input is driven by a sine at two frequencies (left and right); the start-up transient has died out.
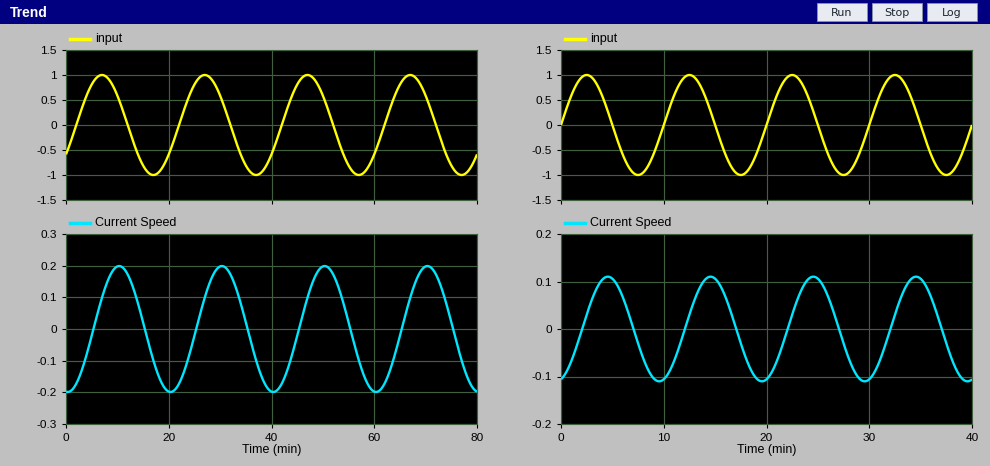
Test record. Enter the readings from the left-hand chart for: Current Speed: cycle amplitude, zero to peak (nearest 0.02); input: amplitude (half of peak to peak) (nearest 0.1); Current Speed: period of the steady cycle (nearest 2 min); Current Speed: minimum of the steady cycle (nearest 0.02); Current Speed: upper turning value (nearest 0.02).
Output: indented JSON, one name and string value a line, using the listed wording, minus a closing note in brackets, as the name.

{
  "Current Speed: cycle amplitude, zero to peak": "0.20",
  "input: amplitude (half of peak to peak)": "1.0",
  "Current Speed: period of the steady cycle": "20 min",
  "Current Speed: minimum of the steady cycle": "-0.20",
  "Current Speed: upper turning value": "0.20"
}
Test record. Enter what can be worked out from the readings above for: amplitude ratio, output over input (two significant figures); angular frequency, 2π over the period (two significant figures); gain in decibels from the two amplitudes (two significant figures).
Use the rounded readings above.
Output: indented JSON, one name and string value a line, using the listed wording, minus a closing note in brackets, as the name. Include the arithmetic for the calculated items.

{
  "amplitude ratio, output over input": "0.2 / 1 = 0.20",
  "angular frequency, 2π over the period": "2π / 20 = 0.31 rad/min",
  "gain in decibels from the two amplitudes": "20 log10(0.2 / 1) = -14 dB"
}
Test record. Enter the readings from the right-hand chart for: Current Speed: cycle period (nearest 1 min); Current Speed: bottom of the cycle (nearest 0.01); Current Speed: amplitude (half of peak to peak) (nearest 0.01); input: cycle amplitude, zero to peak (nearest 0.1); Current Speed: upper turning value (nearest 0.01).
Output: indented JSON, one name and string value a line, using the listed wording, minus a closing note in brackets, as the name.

{
  "Current Speed: cycle period": "10 min",
  "Current Speed: bottom of the cycle": "-0.11",
  "Current Speed: amplitude (half of peak to peak)": "0.11",
  "input: cycle amplitude, zero to peak": "1.0",
  "Current Speed: upper turning value": "0.11"
}
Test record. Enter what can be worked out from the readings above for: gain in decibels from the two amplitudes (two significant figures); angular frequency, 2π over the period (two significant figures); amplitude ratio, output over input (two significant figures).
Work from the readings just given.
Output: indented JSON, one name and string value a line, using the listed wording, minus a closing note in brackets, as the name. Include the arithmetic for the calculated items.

{
  "gain in decibels from the two amplitudes": "20 log10(0.11 / 1) = -19 dB",
  "angular frequency, 2π over the period": "2π / 10 = 0.63 rad/min",
  "amplitude ratio, output over input": "0.11 / 1 = 0.11"
}
